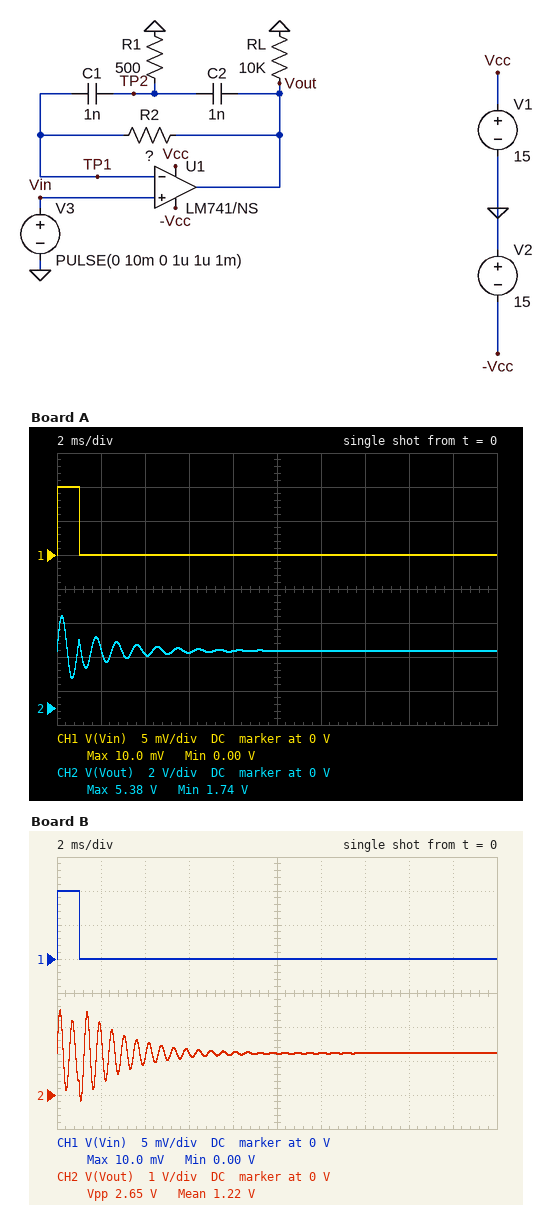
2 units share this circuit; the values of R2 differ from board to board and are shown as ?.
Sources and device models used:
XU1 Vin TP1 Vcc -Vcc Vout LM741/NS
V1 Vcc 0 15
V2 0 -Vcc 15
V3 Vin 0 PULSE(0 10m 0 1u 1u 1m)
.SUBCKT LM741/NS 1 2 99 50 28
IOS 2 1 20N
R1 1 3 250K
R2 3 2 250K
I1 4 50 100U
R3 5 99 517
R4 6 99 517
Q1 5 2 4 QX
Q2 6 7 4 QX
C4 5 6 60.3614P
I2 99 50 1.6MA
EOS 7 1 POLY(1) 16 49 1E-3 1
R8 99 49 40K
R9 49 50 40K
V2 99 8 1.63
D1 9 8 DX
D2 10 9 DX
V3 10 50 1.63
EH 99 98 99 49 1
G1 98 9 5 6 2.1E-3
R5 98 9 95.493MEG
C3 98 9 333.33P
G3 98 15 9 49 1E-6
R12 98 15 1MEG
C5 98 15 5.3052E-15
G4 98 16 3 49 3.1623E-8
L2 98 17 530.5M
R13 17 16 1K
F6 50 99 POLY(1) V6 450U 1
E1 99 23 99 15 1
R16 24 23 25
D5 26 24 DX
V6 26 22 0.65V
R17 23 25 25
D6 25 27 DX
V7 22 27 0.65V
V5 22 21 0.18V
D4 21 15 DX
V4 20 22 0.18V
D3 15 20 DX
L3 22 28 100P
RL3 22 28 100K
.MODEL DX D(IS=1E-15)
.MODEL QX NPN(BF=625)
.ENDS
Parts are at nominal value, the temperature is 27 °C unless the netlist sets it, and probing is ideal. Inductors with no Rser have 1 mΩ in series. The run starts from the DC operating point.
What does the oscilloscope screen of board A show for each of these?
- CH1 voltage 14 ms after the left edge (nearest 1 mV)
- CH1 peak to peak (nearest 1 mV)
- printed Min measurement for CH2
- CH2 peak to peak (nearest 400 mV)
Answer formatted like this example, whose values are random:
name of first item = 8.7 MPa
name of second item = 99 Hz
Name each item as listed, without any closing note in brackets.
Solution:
CH1 voltage 14 ms after the left edge = 0 V
CH1 peak to peak = 10 mV
printed Min measurement for CH2 = 1.74 V
CH2 peak to peak = 3.6 V
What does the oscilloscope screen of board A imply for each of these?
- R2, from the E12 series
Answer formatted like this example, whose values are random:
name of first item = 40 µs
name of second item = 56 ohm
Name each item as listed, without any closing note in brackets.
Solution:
R2, from the E12 series = 33 MΩ
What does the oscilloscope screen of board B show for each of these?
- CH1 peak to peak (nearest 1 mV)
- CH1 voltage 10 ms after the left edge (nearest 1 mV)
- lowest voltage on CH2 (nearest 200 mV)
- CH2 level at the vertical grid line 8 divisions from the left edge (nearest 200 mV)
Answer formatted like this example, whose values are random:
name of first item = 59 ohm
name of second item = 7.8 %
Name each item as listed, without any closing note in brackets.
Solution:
CH1 peak to peak = 10 mV
CH1 voltage 10 ms after the left edge = 0 V
lowest voltage on CH2 = -200 mV
CH2 level at the vertical grid line 8 divisions from the left edge = 1.2 V
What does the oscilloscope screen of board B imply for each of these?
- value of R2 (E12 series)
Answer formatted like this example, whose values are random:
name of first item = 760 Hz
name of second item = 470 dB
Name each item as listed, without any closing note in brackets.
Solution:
value of R2 = 12 MΩ
